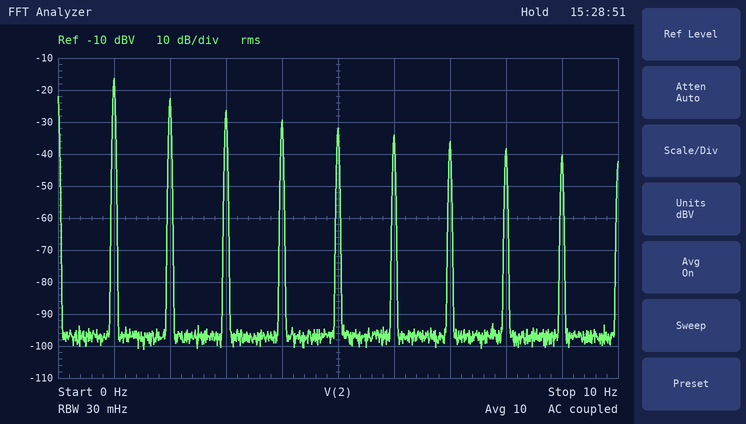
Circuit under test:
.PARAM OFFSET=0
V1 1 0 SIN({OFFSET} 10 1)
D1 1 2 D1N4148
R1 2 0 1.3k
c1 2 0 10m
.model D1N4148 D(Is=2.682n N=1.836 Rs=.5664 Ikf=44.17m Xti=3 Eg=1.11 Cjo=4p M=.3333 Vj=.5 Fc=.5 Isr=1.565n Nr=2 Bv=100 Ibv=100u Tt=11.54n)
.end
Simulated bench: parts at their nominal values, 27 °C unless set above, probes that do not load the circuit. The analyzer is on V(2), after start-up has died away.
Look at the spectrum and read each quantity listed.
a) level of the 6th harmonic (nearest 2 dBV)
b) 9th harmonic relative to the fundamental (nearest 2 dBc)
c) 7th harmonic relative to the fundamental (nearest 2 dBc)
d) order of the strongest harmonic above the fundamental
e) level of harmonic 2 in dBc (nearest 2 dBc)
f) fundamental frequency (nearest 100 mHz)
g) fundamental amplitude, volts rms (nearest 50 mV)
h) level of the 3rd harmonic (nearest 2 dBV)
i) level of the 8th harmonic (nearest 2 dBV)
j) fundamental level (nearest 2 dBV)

-34 dBV
-24 dBc
-20 dBc
2
-6 dBc
1.0 Hz
150 mV
-26 dBV
-38 dBV
-16 dBV
